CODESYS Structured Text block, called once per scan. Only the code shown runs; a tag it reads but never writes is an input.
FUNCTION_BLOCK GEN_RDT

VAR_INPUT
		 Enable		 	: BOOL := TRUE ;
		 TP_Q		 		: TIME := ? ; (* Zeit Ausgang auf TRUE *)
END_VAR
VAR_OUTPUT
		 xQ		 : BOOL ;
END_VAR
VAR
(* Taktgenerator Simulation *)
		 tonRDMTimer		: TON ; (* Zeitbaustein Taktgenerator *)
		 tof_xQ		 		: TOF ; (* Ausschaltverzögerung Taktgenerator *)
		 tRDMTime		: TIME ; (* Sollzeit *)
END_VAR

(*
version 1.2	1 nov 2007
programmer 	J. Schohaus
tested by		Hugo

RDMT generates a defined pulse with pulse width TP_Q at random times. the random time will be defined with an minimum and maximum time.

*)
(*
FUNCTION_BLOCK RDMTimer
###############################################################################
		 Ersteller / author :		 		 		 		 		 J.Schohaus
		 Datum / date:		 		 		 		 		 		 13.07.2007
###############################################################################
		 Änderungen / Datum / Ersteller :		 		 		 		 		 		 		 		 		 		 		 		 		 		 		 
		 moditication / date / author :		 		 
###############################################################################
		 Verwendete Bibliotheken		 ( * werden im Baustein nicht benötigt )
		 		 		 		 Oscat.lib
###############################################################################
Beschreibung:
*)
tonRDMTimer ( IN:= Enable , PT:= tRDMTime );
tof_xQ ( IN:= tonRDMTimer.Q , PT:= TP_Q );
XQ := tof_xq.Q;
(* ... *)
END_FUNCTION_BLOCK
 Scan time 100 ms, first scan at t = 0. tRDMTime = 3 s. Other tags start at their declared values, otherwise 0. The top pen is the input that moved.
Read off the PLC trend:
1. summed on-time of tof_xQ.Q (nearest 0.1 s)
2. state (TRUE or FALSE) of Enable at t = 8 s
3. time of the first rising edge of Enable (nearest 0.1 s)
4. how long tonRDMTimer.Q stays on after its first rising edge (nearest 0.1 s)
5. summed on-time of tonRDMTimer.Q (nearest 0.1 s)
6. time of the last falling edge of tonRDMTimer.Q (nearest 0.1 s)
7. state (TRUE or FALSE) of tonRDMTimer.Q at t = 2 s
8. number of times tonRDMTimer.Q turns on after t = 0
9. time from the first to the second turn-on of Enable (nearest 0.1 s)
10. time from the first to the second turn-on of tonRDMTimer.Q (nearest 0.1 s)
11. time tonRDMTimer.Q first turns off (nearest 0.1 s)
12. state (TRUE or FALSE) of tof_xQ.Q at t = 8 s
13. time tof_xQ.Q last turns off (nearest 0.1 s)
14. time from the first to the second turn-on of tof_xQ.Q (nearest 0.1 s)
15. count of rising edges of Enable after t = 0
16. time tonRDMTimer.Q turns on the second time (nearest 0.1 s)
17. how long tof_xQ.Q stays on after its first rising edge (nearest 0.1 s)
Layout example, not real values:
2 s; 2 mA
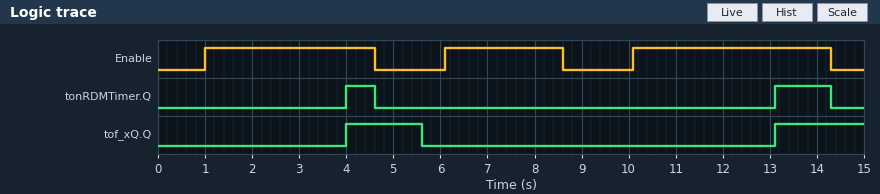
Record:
3.5 s; TRUE; 1.0 s; 0.6 s; 1.8 s; 14.3 s; FALSE; 2; 5.1 s; 9.1 s; 4.6 s; FALSE; 5.6 s; 9.1 s; 3; 13.1 s; 1.6 s
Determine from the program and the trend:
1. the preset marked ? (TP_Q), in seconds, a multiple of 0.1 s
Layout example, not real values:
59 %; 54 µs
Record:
1.0 s
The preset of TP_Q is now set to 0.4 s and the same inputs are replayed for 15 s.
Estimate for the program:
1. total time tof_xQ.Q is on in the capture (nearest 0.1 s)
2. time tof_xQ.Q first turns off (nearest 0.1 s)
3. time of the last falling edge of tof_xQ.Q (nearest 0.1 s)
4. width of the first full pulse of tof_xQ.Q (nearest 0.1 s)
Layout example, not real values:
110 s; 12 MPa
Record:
2.6 s; 5.0 s; 14.7 s; 1.0 s
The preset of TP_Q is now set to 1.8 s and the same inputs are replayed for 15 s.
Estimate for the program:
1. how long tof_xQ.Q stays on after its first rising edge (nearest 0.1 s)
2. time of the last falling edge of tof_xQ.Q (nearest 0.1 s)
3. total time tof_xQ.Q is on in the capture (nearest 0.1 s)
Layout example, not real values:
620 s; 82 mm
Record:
2.4 s; 6.4 s; 4.3 s
